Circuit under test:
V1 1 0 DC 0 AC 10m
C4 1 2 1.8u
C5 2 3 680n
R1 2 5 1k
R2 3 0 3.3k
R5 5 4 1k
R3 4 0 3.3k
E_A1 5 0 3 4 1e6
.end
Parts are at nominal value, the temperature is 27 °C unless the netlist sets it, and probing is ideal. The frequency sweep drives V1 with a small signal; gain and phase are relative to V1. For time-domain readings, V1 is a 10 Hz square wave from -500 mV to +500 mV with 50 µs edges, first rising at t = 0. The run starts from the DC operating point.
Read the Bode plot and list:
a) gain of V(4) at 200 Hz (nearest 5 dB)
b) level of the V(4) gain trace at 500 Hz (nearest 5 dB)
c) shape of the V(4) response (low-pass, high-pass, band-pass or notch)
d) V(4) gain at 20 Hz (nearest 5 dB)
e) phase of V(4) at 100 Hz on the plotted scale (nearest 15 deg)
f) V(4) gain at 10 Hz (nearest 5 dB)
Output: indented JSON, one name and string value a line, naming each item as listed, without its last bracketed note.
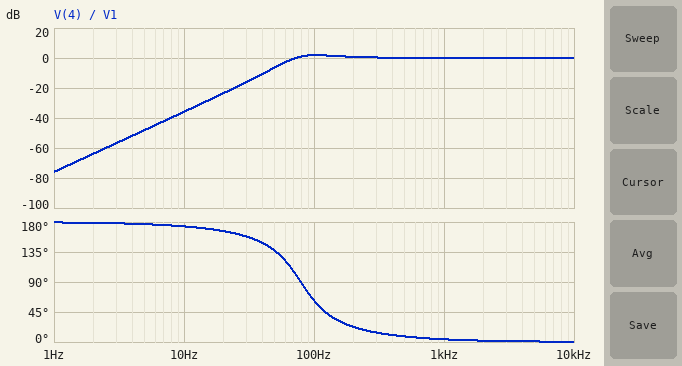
{
  "gain of V(4) at 200 Hz": "0 dB",
  "level of the V(4) gain trace at 500 Hz": "0 dB",
  "shape of the V(4) response": "high-pass",
  "V(4) gain at 20 Hz": "-25 dB",
  "phase of V(4) at 100 Hz on the plotted scale": "60 deg",
  "V(4) gain at 10 Hz": "-35 dB"
}
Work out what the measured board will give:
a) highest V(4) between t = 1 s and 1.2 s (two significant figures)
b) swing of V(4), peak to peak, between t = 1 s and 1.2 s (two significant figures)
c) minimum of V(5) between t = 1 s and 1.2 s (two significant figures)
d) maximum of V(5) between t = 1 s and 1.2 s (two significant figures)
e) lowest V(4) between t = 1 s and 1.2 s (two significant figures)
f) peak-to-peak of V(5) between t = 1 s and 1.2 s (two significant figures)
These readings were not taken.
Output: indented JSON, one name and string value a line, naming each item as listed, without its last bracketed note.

{
  "highest V(4) between t = 1 s and 1.2 s": "990 mV",
  "swing of V(4), peak to peak, between t = 1 s and 1.2 s": "2.0 V",
  "minimum of V(5) between t = 1 s and 1.2 s": "-1.3 V",
  "maximum of V(5) between t = 1 s and 1.2 s": "1.3 V",
  "lowest V(4) between t = 1 s and 1.2 s": "-990 mV",
  "peak-to-peak of V(5) between t = 1 s and 1.2 s": "2.6 V"
}
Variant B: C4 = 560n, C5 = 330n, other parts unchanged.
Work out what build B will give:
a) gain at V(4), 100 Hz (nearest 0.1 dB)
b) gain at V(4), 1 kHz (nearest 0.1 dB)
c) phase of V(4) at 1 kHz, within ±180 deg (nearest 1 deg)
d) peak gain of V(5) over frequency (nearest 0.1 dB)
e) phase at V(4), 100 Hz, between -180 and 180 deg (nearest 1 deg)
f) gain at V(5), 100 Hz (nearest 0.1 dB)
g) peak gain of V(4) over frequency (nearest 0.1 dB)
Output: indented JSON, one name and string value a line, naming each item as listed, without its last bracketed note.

{
  "gain at V(4), 100 Hz": "-10.8 dB",
  "gain at V(4), 1 kHz": "0.3 dB",
  "phase of V(4) at 1 kHz, within ±180 deg": "9 deg",
  "peak gain of V(5) over frequency": "5.8 dB",
  "phase at V(4), 100 Hz, between -180 and 180 deg": "155 deg",
  "gain at V(5), 100 Hz": "-8.5 dB",
  "peak gain of V(4) over frequency": "3.5 dB"
}
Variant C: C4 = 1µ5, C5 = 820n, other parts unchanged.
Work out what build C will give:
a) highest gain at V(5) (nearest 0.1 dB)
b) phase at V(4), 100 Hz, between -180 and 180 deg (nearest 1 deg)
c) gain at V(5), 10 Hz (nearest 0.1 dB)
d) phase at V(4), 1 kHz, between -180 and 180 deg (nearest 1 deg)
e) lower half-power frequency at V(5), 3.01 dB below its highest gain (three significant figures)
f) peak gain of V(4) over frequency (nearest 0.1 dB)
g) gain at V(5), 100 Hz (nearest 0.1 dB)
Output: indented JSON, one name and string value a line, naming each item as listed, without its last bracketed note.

{
  "highest gain at V(5)": "5.5 dB",
  "phase at V(4), 100 Hz, between -180 and 180 deg": "57 deg",
  "gain at V(5), 10 Hz": "-33.5 dB",
  "phase at V(4), 1 kHz, between -180 and 180 deg": "3 deg",
  "lower half-power frequency at V(5), 3.01 dB below its highest gain": "66.4 Hz",
  "peak gain of V(4) over frequency": "3.2 dB",
  "gain at V(5), 100 Hz": "5.4 dB"
}
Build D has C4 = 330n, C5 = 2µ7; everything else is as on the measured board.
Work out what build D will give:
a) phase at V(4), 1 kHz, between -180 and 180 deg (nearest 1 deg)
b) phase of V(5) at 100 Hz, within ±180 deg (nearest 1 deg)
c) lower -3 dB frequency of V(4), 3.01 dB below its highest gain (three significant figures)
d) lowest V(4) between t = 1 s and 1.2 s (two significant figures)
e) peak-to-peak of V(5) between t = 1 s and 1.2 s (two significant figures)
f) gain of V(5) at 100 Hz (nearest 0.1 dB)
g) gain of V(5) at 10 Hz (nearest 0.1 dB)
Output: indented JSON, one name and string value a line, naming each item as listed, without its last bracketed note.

{
  "phase at V(4), 1 kHz, between -180 and 180 deg": "1 deg",
  "phase of V(5) at 100 Hz, within ±180 deg": "52 deg",
  "lower -3 dB frequency of V(4), 3.01 dB below its highest gain": "85.7 Hz",
  "lowest V(4) between t = 1 s and 1.2 s": "-1.0 V",
  "peak-to-peak of V(5) between t = 1 s and 1.2 s": "2.7 V",
  "gain of V(5) at 100 Hz": "15.2 dB",
  "gain of V(5) at 10 Hz": "-36.3 dB"
}
